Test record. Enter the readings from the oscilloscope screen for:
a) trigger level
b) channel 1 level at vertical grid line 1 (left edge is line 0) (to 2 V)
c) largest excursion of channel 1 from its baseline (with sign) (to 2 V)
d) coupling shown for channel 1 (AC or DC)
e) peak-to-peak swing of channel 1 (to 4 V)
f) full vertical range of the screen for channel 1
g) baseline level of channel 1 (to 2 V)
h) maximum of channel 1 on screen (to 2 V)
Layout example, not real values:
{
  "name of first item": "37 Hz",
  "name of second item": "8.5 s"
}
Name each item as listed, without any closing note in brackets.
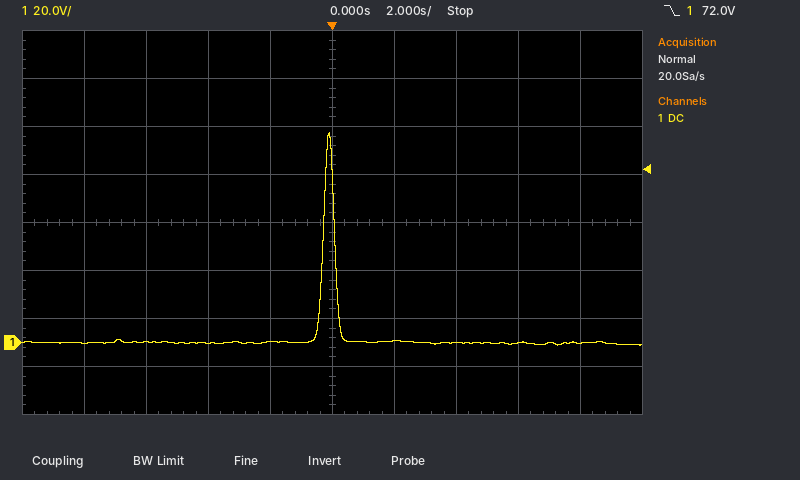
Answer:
{
  "trigger level": "72.0 V",
  "channel 1 level at vertical grid line 1 (left edge is line 0)": "0 V",
  "largest excursion of channel 1 from its baseline (with sign)": "+88 V",
  "coupling shown for channel 1": "DC",
  "peak-to-peak swing of channel 1": "88 V",
  "full vertical range of the screen for channel 1": "160 V",
  "baseline level of channel 1": "0 V",
  "maximum of channel 1 on screen": "88 V"
}
